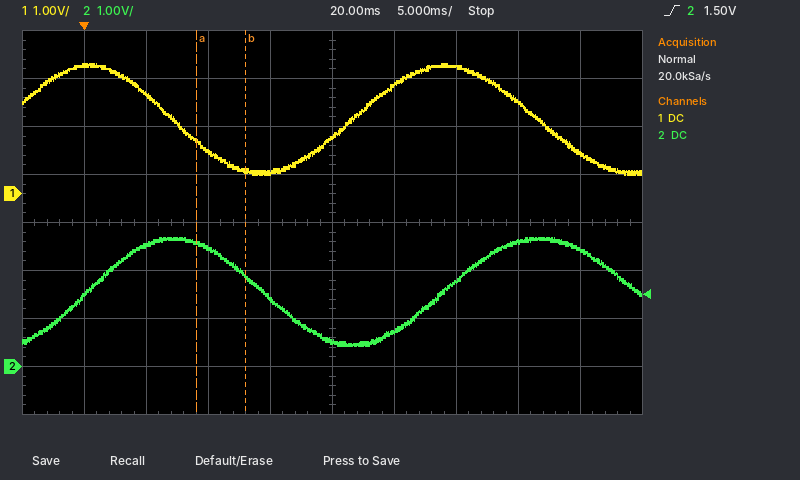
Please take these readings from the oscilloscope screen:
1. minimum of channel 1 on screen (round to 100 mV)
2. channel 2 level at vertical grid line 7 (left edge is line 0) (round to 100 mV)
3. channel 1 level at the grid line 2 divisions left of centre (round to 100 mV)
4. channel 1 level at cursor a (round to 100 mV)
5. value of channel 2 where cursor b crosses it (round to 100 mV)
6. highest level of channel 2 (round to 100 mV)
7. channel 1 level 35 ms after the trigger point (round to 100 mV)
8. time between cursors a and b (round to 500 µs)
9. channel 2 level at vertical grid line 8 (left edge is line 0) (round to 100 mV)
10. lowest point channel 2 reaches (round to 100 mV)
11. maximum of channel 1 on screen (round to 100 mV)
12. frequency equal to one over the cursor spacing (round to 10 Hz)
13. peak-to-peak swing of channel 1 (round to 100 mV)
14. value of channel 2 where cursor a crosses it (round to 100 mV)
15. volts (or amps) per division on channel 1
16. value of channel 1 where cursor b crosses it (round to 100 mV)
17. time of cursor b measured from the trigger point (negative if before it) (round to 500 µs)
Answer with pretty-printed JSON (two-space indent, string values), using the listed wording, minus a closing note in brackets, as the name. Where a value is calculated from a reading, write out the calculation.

{
  "minimum of channel 1 on screen": "400 mV",
  "channel 2 level at vertical grid line 7 (left edge is line 0)": "1.8 V",
  "channel 1 level at the grid line 2 divisions left of centre": "900 mV",
  "channel 1 level at cursor a": "1.1 V",
  "value of channel 2 where cursor b crosses it": "1.9 V",
  "highest level of channel 2": "2.7 V",
  "channel 1 level 35 ms after the trigger point": "1.9 V",
  "time between cursors a and b": "4.0 ms",
  "channel 2 level at vertical grid line 8 (left edge is line 0)": "2.6 V",
  "lowest point channel 2 reaches": "400 mV",
  "maximum of channel 1 on screen": "2.7 V",
  "frequency equal to one over the cursor spacing": "1 / 4.0 ms ≈ 250 Hz",
  "peak-to-peak swing of channel 1": "2.7 V − (400 mV) = 2.3 V",
  "value of channel 2 where cursor a crosses it": "2.6 V",
  "volts (or amps) per division on channel 1": "1 V",
  "value of channel 1 where cursor b crosses it": "500 mV",
  "time of cursor b measured from the trigger point (negative if before it)": "+13.0 ms"
}
